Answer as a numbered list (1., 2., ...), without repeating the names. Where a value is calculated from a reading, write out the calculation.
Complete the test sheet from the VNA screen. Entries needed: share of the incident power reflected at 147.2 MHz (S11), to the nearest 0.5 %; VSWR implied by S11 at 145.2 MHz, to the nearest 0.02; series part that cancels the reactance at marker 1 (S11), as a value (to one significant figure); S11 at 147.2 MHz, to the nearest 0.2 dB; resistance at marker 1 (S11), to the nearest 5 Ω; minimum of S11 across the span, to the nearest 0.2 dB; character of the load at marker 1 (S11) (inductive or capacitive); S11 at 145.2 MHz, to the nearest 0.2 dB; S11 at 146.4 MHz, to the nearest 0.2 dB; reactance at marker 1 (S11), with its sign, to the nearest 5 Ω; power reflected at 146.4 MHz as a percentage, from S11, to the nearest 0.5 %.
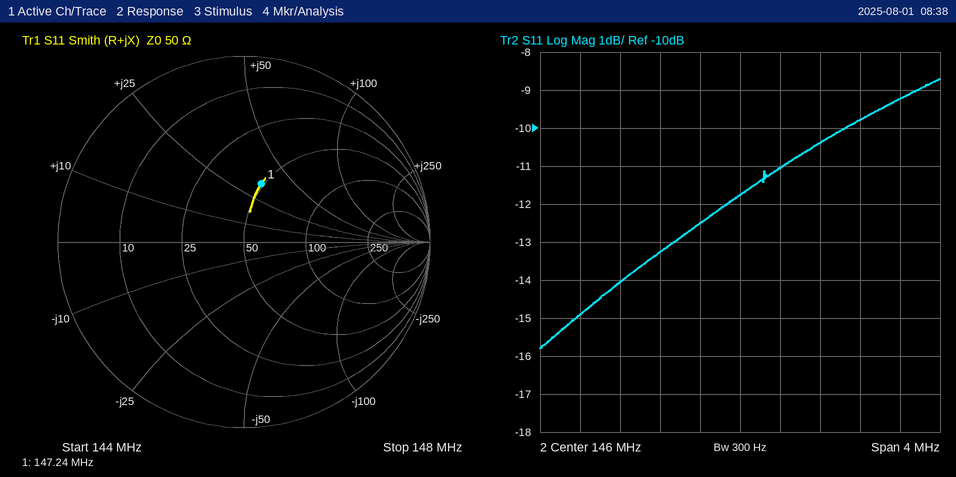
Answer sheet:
1. 10^(-9.8/10) ≈ 10.5 %
2. |Γ| = 10^(-13.2/20) = 0.2188; VSWR = (1 + 0.2188)/(1 − 0.2188) ≈ 1.56
3. C = 1/(2π × 147.24 MHz × 35 Ω) ≈ 30.9 pF, so 30 pF to one significant figure
4. -9.8 dB
5. 50 Ω
6. -15.8 dB
7. inductive
8. -13.2 dB
9. -11.0 dB
10. +35 Ω
11. 10^(-11/10) ≈ 7.94 %, so 8.0 % to the nearest 0.5 %
